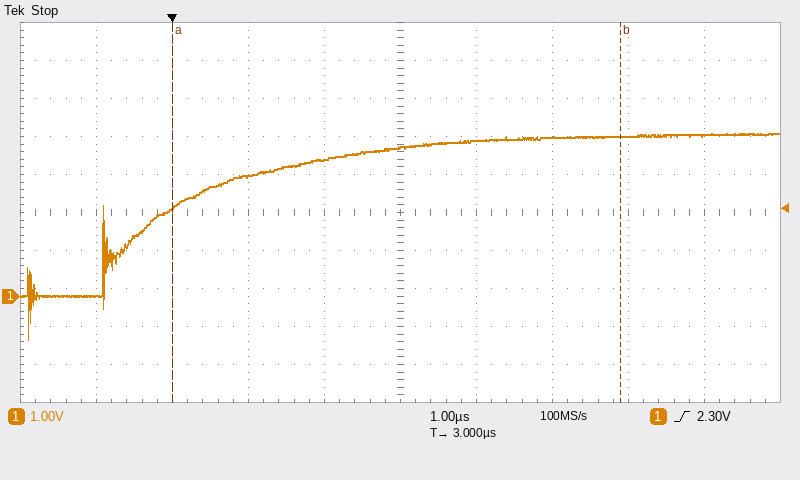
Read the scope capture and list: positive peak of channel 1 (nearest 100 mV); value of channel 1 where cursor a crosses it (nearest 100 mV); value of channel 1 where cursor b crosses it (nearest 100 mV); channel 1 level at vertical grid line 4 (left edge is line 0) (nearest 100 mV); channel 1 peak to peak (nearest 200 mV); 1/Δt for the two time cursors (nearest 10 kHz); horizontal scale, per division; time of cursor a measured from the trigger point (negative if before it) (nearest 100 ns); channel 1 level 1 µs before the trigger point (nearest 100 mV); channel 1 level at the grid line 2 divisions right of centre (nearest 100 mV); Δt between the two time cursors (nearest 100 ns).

4.3 V
2.3 V
4.2 V
3.6 V
5.4 V
170 kHz
1 µs
0.0 µs
0.0 V
4.2 V
5.9 µs
